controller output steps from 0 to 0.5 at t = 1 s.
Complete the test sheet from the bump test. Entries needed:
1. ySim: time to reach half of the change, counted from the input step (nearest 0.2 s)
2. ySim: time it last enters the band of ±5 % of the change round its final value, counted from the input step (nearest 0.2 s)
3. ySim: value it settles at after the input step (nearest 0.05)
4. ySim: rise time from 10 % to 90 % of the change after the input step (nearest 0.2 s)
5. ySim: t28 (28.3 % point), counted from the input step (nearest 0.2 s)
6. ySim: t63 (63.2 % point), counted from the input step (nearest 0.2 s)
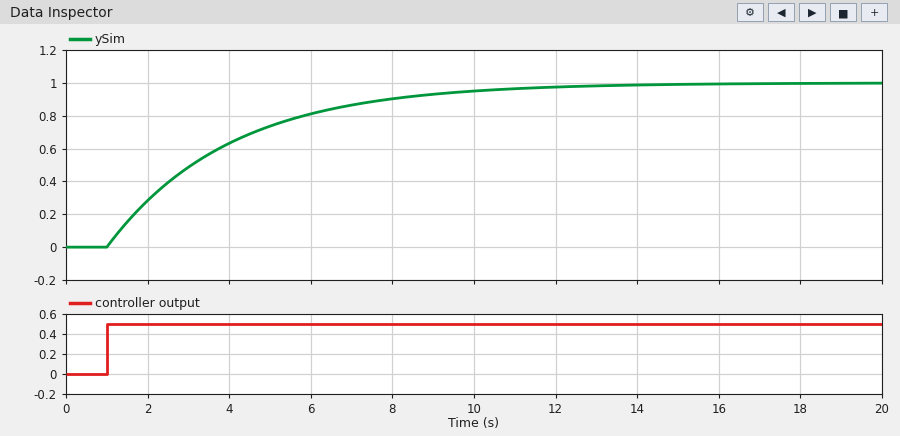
2.0 s
9.0 s
1.00
6.6 s
1.0 s
3.0 s
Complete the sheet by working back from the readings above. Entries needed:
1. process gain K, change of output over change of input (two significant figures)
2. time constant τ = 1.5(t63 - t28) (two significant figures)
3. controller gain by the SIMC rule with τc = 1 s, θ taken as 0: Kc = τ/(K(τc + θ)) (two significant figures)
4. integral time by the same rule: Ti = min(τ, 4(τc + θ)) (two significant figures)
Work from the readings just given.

2.0
3.0 s
1.5
3.0 s
